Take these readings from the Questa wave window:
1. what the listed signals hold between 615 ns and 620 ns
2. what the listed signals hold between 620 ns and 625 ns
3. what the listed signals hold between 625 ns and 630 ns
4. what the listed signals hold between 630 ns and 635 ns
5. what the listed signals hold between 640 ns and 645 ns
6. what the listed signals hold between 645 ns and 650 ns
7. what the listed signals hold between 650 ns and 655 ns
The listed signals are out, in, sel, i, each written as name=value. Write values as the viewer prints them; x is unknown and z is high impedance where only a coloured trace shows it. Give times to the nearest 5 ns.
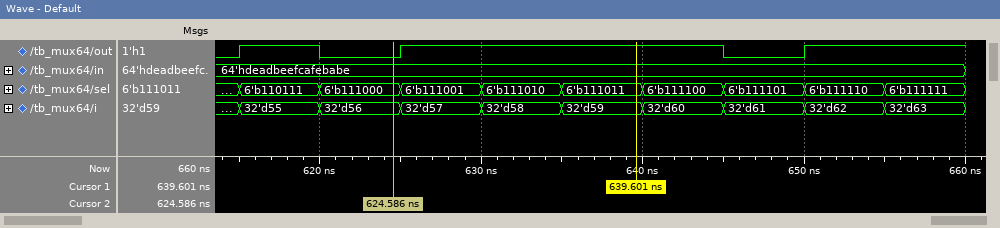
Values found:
out=1, in=64'hdeadbeefcafebabe, sel=6'b110111, i=32'd55
out=0, in=64'hdeadbeefcafebabe, sel=6'b111000, i=32'd56
out=1, in=64'hdeadbeefcafebabe, sel=6'b111001, i=32'd57
out=1, in=64'hdeadbeefcafebabe, sel=6'b111010, i=32'd58
out=1, in=64'hdeadbeefcafebabe, sel=6'b111100, i=32'd60
out=0, in=64'hdeadbeefcafebabe, sel=6'b111101, i=32'd61
out=1, in=64'hdeadbeefcafebabe, sel=6'b111110, i=32'd62
